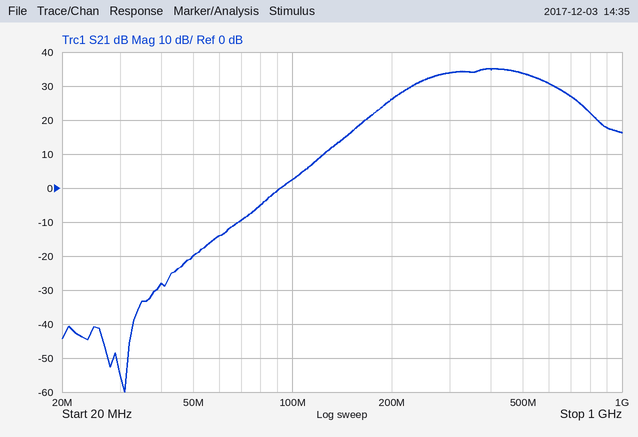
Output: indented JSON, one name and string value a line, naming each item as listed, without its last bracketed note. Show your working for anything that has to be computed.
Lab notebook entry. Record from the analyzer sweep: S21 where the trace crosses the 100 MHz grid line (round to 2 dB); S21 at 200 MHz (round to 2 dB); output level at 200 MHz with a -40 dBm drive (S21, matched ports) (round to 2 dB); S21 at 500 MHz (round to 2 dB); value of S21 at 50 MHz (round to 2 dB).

{
  "S21 where the trace crosses the 100 MHz grid line": "2 dB",
  "S21 at 200 MHz": "26 dB",
  "output level at 200 MHz with a -40 dBm drive (S21, matched ports)": "-40 dBm + (26 dB) = -14 dBm",
  "S21 at 500 MHz": "34 dB",
  "value of S21 at 50 MHz": "-20 dB"
}
